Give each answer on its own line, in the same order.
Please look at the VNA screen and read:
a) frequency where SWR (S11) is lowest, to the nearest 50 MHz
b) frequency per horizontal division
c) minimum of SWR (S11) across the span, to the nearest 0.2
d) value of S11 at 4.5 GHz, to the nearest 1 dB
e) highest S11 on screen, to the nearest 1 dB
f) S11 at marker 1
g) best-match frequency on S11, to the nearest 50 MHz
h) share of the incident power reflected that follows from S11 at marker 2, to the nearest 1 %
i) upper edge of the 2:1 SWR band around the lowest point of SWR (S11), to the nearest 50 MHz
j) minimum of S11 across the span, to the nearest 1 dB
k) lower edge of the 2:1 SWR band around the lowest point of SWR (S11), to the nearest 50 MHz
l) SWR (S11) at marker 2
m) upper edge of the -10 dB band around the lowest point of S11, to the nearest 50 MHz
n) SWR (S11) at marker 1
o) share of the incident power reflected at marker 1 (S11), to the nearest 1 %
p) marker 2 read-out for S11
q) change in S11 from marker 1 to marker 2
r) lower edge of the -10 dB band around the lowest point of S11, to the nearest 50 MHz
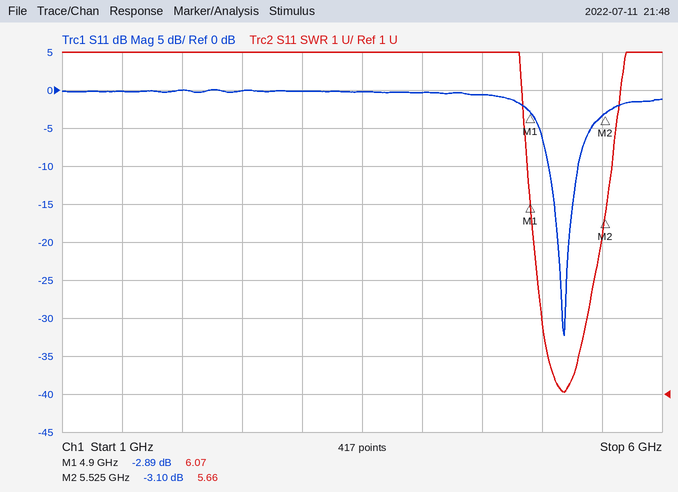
5.20 GHz
500 MHz
1.0
-1 dB
0 dB
-2.89 dB
5.20 GHz
49 %
5.30 GHz
-32 dB
5.05 GHz
5.66
5.30 GHz
6.07
51 %
-3.10 dB
-0.21 dB
5.05 GHz
